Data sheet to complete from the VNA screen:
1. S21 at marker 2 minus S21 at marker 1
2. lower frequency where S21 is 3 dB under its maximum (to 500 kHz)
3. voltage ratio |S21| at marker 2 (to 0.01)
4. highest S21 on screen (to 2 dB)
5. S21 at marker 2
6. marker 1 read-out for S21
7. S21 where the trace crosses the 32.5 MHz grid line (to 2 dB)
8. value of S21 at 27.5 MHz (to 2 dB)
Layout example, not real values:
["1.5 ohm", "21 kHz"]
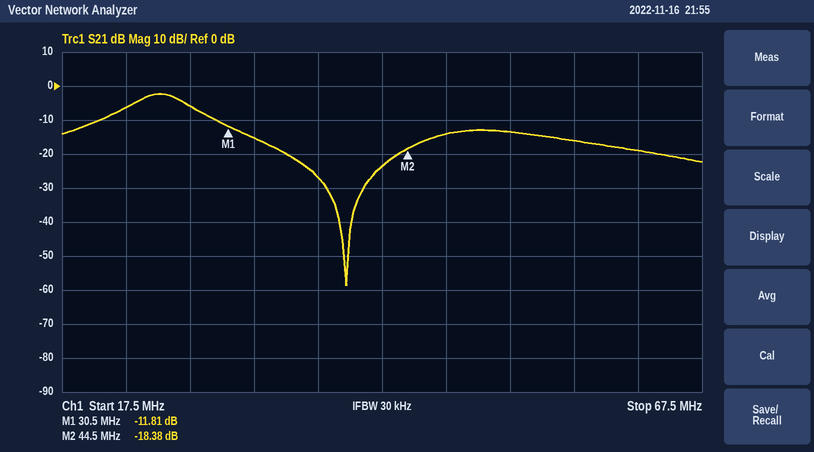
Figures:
["-6.57 dB", "23.0 MHz", "0.12", "-2 dB", "-18.38 dB", "-11.81 dB", "-16 dB", "-6 dB"]
